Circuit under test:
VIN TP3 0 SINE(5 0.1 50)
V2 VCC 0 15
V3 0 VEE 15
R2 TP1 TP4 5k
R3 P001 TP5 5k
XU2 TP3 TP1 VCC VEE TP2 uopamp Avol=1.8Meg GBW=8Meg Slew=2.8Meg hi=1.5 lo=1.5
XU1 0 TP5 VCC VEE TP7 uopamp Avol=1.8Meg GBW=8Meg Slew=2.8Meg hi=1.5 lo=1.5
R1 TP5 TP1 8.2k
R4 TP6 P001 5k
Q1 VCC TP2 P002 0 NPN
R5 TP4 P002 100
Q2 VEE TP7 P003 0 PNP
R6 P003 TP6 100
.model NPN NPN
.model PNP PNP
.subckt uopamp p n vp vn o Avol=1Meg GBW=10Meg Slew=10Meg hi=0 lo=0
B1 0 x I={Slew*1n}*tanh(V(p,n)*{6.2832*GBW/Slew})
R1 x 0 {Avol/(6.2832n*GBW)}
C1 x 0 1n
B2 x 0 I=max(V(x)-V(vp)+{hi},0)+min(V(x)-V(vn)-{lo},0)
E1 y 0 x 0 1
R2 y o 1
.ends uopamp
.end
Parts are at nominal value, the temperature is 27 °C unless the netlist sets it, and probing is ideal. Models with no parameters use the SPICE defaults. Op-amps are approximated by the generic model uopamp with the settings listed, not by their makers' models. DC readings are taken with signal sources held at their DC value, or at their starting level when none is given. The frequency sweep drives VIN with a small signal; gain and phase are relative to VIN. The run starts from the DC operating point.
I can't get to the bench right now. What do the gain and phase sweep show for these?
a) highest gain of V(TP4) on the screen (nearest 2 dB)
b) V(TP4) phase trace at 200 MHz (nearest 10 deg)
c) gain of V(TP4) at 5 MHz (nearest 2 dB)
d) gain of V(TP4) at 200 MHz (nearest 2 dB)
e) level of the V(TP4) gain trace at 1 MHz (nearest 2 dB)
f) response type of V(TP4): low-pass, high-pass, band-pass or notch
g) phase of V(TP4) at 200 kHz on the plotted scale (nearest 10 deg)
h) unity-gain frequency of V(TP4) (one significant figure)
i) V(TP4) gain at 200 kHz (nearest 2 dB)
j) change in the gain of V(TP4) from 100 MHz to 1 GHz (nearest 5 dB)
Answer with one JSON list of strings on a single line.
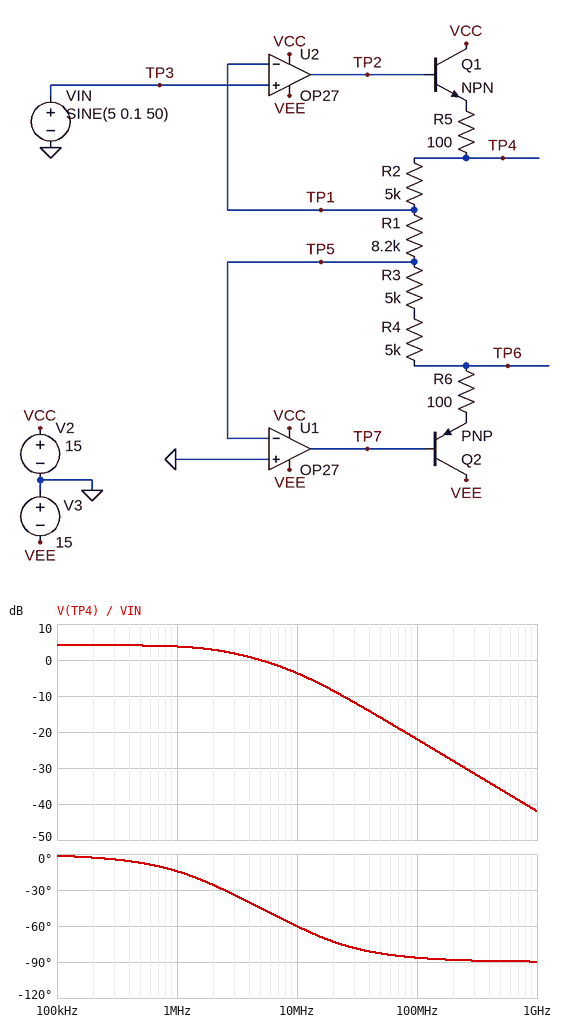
["4 dB", "-90 deg", "0 dB", "-28 dB", "4 dB", "low-pass", "0 deg", "5 MHz", "4 dB", "-20 dB"]
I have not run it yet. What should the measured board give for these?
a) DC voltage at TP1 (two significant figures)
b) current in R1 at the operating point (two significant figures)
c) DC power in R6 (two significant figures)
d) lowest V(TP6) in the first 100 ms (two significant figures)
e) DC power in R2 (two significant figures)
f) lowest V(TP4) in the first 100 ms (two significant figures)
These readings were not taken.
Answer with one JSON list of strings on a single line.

["5.0 V", "610 µA", "37 µW", "-6.2 V", "1.9 mW", "7.9 V"]
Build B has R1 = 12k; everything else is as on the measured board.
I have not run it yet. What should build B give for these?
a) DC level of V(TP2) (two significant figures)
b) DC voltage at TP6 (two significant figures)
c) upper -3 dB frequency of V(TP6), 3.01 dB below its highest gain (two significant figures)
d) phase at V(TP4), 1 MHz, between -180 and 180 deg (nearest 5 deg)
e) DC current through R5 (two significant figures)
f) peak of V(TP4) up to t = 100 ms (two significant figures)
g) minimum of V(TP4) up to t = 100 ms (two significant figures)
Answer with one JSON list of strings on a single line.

["7.9 V", "-4.2 V", "3.0 MHz", "-10 deg", "420 µA", "7.2 V", "6.9 V"]
